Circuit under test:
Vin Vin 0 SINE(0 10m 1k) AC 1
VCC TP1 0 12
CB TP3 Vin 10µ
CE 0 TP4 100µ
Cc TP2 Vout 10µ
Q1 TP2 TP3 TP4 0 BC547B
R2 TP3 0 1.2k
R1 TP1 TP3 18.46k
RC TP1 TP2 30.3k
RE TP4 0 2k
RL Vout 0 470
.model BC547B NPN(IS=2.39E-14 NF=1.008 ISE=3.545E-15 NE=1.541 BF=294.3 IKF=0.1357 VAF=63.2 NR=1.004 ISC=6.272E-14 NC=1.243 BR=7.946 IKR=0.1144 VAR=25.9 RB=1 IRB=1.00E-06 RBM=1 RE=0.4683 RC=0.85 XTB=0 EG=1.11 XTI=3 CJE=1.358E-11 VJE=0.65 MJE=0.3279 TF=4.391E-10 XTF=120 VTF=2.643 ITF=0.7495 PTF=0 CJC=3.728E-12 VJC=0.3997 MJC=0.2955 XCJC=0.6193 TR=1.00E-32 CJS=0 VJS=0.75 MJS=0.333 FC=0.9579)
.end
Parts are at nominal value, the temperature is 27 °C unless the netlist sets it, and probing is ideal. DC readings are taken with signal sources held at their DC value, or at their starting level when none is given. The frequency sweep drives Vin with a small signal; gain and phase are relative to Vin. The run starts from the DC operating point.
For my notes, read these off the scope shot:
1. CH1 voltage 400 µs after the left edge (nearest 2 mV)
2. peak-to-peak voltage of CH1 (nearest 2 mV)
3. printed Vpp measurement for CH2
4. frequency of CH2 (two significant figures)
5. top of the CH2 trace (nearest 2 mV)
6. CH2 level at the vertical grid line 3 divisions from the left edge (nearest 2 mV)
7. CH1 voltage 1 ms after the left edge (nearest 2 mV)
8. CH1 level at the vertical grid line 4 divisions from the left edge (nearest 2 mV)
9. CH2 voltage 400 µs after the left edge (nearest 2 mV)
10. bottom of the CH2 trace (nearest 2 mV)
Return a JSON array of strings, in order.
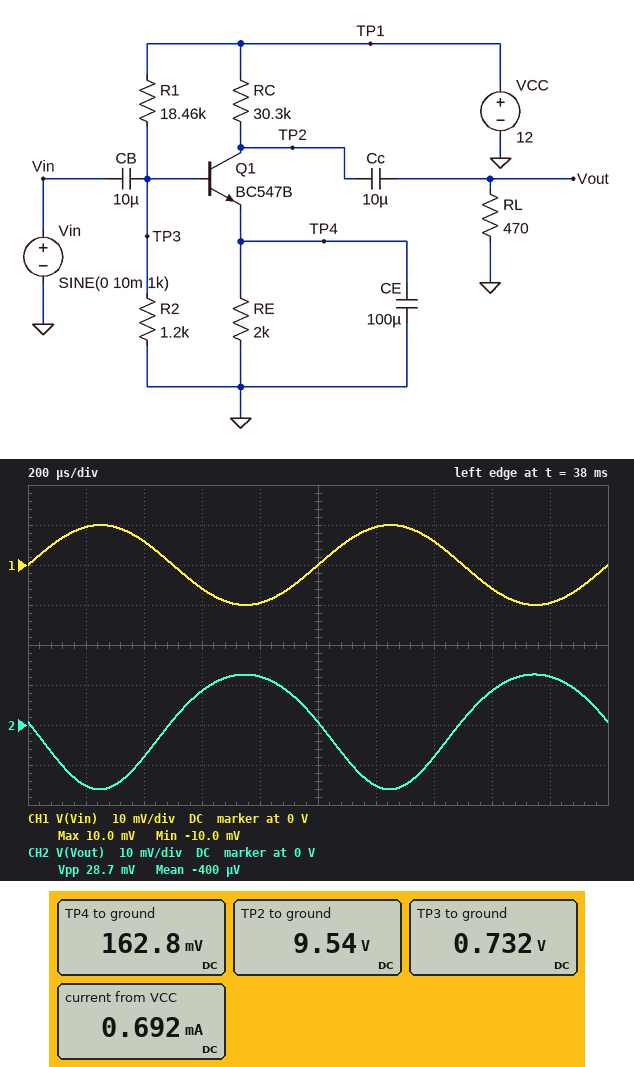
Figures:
["6 mV", "20 mV", "28.7 mV", "1.0 kHz", "12 mV", "8 mV", "0 V", "-10 mV", "-8 mV", "-16 mV"]
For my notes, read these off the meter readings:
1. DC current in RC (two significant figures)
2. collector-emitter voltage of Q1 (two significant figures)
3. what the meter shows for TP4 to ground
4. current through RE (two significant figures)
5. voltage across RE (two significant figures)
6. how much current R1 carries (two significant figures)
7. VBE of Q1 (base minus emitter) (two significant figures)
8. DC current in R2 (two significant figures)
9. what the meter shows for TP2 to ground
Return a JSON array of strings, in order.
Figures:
["81 µA", "9.4 V", "162.8 mV", "81 µA", "160 mV", "610 µA", "570 mV", "610 µA", "9.54 V"]
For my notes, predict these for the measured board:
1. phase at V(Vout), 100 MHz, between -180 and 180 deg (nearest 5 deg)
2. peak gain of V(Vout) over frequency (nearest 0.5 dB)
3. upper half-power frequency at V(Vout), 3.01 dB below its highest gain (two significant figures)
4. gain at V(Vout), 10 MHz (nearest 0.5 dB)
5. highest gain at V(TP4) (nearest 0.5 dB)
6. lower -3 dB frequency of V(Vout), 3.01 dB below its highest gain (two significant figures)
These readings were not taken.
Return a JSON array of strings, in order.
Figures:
["140 deg", "3.0 dB", "1.4 GHz", "3.0 dB", "-12.0 dB", "16 Hz"]
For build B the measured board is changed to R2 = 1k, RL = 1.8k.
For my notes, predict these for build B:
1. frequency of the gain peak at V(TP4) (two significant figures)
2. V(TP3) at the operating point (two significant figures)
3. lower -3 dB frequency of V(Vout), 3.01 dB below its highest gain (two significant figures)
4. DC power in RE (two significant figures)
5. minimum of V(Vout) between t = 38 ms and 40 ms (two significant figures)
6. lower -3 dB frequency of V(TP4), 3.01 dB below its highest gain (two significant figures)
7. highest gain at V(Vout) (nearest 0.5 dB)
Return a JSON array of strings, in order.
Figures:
["7.0 Hz", "620 mV", "17 Hz", "2.4 µW", "-26 mV", "2.2 Hz", "7.0 dB"]
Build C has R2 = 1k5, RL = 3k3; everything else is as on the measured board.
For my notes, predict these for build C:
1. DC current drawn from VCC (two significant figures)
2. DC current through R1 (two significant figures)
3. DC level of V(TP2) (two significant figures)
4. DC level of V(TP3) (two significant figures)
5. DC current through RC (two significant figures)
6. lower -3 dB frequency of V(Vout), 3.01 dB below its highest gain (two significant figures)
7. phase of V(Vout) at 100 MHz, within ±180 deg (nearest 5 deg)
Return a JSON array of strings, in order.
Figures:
["760 µA", "600 µA", "7.3 V", "900 mV", "160 µA", "17 Hz", "95 deg"]
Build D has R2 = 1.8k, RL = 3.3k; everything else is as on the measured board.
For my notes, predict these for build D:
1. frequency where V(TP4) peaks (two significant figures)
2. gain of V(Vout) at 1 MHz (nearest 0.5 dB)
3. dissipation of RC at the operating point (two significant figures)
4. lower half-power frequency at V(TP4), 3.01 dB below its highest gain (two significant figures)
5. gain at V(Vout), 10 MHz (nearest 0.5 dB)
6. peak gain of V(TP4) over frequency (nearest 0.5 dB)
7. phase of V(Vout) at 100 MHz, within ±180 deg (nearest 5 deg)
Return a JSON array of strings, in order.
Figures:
["12 Hz", "28.5 dB", "1.6 mW", "4.8 Hz", "28.0 dB", "-5.0 dB", "95 deg"]
